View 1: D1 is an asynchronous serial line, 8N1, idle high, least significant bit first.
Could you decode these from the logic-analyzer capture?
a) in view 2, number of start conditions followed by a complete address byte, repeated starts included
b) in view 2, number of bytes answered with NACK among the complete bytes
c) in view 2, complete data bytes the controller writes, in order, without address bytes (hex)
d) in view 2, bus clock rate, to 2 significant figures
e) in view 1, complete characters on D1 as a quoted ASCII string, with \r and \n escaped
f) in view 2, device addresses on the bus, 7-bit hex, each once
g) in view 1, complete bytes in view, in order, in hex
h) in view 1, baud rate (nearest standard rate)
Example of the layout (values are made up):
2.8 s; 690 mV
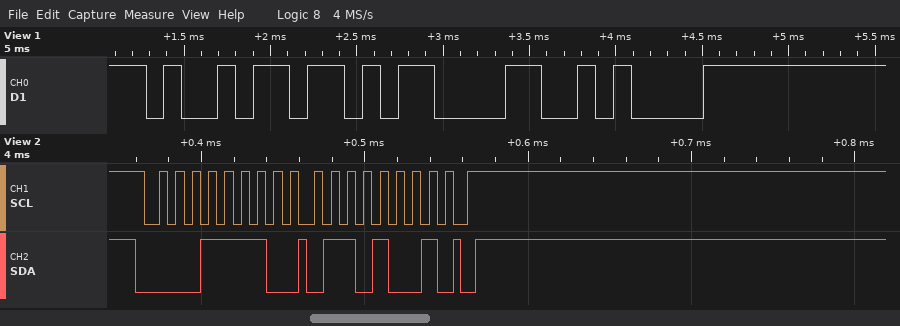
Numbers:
1; 0; 69; 100 kHz; "i\r\n"; 0x0F; 69 0D 0A; 9600 baud
